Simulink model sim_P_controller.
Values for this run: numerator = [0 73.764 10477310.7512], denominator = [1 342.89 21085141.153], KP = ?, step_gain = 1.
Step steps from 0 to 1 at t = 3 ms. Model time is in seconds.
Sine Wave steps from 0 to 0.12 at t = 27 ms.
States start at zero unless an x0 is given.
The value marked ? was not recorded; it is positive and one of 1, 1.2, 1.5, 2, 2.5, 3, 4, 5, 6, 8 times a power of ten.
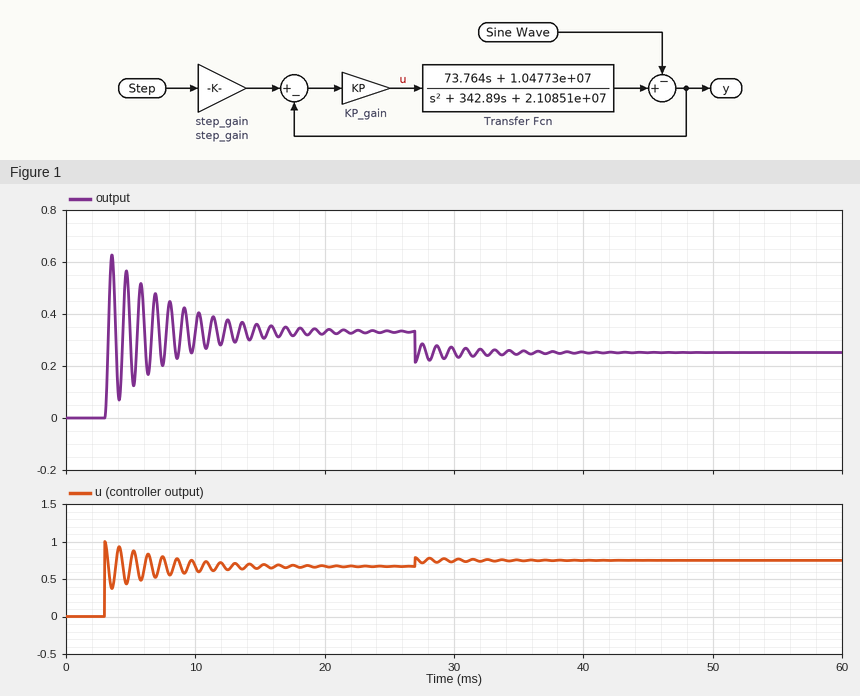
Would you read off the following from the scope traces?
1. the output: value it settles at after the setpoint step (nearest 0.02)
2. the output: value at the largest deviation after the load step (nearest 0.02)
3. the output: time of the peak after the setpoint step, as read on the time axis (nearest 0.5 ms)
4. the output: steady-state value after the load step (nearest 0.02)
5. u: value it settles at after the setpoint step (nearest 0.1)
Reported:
0.34
0.22
3.5 ms
0.26
0.7
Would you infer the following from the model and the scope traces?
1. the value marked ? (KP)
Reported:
1
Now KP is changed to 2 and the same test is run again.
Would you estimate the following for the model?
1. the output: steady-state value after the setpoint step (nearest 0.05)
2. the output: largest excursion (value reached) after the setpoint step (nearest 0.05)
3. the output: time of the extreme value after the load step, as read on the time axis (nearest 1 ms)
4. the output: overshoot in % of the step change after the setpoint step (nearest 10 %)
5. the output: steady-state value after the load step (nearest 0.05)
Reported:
0.50
0.95
27 ms
90 %
0.45
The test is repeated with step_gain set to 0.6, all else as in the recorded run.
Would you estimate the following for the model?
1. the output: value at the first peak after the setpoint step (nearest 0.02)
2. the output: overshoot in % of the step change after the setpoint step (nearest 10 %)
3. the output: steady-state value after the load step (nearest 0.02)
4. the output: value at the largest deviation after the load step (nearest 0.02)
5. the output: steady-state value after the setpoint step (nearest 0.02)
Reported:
0.38
90 %
0.12
0.08
0.20
